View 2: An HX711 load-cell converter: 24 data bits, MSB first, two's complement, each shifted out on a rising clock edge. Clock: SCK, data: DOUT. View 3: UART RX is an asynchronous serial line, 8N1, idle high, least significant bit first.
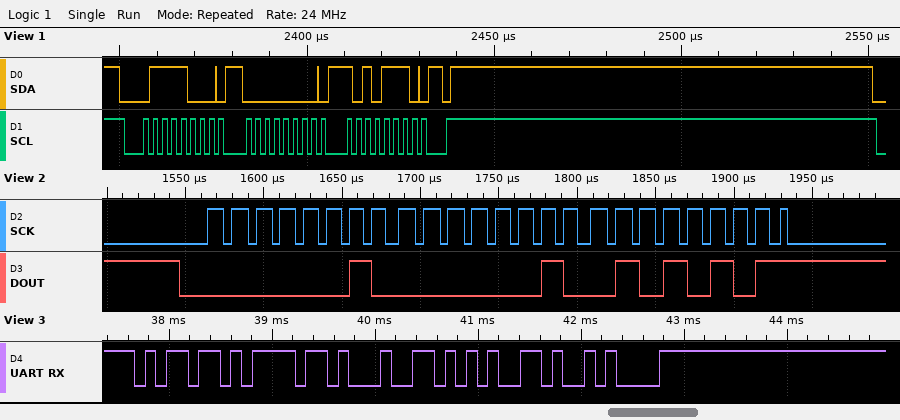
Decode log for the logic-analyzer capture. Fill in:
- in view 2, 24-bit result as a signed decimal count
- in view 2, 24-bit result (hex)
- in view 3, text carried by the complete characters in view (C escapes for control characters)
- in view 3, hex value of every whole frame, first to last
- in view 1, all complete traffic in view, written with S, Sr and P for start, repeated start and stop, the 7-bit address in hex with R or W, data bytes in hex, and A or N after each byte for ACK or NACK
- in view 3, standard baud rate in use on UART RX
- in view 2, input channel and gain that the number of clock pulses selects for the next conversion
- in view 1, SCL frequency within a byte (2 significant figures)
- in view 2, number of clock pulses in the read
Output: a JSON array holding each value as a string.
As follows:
["131669", "0x020255", "\"mode\\n\"", "6D 6F 64 65 0A", "S 3CW A 00 A AE A P", "9600 baud", "channel A, gain 128", "400 kHz", "25"]
